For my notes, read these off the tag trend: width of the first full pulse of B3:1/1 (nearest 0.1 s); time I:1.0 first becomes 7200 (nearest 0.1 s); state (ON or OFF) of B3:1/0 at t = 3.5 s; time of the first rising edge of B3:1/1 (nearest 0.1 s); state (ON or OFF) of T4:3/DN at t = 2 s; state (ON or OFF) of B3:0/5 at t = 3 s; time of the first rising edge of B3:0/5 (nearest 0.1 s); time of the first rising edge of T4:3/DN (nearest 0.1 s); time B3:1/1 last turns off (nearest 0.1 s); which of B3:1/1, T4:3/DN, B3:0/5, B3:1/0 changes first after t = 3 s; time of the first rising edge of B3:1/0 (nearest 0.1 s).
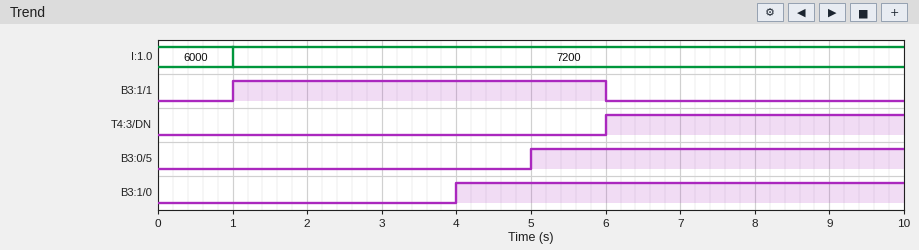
5.0 s
1.0 s
OFF
1.0 s
OFF
OFF
5.0 s
6.0 s
6.0 s
B3:1/0
4.0 s
